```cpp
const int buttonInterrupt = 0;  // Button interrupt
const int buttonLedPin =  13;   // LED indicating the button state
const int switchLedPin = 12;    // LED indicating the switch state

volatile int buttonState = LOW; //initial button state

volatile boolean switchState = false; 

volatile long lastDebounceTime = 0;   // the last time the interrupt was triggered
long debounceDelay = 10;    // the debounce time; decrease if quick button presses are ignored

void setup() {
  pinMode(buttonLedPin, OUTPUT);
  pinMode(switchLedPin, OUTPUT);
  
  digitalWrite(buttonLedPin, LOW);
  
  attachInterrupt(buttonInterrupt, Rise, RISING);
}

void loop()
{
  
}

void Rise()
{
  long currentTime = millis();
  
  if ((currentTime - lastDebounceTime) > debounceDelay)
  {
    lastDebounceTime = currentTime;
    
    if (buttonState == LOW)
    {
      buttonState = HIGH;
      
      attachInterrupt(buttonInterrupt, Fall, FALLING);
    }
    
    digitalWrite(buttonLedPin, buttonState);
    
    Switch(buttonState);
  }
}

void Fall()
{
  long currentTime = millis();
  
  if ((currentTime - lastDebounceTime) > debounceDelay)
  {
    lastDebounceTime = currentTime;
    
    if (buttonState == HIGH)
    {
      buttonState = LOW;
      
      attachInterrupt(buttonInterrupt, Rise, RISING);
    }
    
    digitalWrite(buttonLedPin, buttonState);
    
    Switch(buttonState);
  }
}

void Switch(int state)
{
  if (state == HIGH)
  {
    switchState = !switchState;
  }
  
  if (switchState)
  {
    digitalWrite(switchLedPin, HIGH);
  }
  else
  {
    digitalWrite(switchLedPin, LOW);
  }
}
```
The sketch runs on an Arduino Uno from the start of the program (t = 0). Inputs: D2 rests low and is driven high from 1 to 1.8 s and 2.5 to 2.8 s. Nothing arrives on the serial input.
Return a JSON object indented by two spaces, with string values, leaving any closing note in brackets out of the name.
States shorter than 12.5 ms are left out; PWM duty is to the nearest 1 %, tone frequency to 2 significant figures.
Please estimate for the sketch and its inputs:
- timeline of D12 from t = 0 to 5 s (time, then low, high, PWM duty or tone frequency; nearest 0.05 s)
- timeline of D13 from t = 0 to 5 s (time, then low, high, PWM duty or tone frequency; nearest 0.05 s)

{
  "timeline of D12 from t = 0 to 5 s": "0 s low; 1 s high; 2.5 s low",
  "timeline of D13 from t = 0 to 5 s": "0 s low; 1 s high; 1.8 s low; 2.5 s high; 2.8 s low"
}
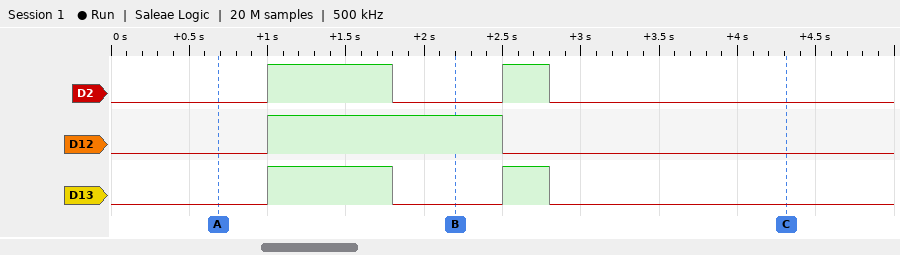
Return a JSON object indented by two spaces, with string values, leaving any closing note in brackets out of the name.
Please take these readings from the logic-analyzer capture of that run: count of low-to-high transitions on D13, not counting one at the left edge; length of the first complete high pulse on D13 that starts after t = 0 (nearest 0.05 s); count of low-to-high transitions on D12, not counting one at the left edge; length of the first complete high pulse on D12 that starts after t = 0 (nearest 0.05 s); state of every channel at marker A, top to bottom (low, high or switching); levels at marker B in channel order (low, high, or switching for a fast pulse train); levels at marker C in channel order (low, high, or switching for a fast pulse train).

{
  "count of low-to-high transitions on D13, not counting one at the left edge": "2",
  "length of the first complete high pulse on D13 that starts after t = 0": "0.80 s",
  "count of low-to-high transitions on D12, not counting one at the left edge": "1",
  "length of the first complete high pulse on D12 that starts after t = 0": "1.50 s",
  "state of every channel at marker A, top to bottom": "D2 low, D12 low, D13 low",
  "levels at marker B in channel order": "D2 low, D12 high, D13 low",
  "levels at marker C in channel order": "D2 low, D12 low, D13 low"
}
